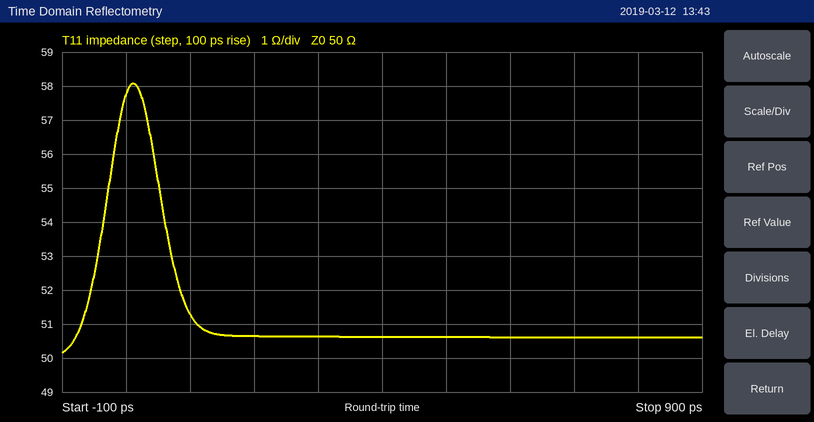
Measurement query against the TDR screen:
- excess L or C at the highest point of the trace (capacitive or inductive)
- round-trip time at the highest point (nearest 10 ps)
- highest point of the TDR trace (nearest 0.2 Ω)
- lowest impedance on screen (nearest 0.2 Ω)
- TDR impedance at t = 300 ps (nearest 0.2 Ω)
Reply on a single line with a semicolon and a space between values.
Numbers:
inductive; 10 ps; 58.0 Ω; 50.2 Ω; 50.6 Ω
